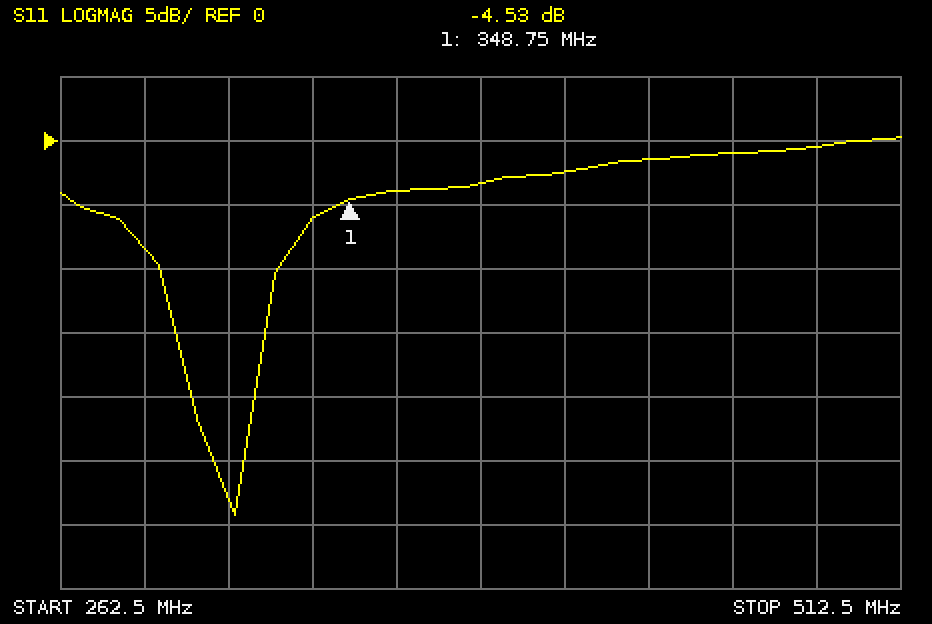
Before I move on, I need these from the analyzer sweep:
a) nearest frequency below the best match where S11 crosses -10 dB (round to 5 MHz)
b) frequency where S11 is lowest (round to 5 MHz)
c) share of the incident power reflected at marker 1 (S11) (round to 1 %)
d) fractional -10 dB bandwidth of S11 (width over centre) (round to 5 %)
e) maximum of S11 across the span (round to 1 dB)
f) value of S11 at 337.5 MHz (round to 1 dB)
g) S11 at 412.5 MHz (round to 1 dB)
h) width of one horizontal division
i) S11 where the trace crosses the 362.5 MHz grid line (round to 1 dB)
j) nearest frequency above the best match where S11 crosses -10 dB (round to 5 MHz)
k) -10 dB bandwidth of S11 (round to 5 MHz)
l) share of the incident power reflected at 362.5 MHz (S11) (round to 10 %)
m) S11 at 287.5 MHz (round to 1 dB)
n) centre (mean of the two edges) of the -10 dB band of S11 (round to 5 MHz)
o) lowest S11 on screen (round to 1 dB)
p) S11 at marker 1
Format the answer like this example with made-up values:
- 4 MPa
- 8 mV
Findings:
- 290 MHz
- 315 MHz
- 35 %
- 10 %
- 0 dB
- -6 dB
- -2 dB
- 25 MHz
- -4 dB
- 325 MHz
- 35 MHz
- 40 %
- -8 dB
- 310 MHz
- -29 dB
- -4.53 dB
